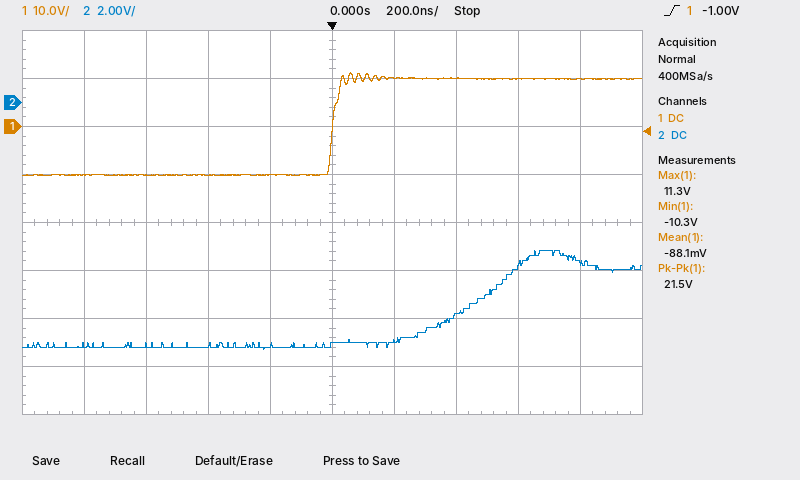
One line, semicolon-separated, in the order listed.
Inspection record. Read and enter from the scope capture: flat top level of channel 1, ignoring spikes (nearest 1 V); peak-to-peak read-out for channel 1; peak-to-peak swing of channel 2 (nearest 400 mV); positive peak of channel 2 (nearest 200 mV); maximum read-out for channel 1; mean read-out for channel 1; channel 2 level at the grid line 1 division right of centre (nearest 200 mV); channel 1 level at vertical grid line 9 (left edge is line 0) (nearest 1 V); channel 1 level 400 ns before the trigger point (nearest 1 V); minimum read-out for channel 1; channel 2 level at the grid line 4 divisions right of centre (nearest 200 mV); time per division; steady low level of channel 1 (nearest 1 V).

10 V; 21.5 V; 4.0 V; -6.2 V; 11.3 V; -88.1 mV; -10.0 V; 10 V; -10 V; -10.3 V; -6.6 V; 200 ns; -10 V
